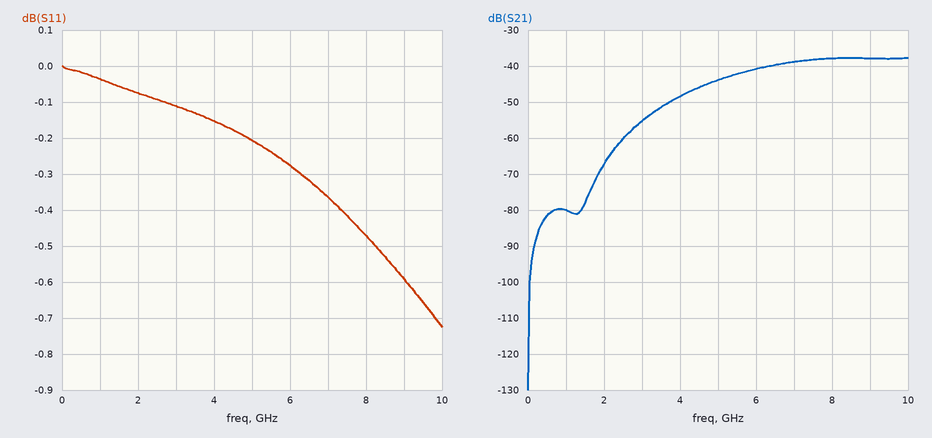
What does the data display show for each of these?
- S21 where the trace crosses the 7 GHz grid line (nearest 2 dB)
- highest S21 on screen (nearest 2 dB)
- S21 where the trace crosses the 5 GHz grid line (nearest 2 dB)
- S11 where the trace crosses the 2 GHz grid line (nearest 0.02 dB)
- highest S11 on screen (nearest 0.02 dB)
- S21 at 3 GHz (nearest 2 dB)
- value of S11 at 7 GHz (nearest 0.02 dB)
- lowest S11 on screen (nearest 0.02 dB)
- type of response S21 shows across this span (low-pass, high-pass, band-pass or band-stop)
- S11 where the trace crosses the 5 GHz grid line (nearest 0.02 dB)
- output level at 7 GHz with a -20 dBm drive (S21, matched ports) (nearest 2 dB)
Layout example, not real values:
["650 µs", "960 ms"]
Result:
["-38 dB", "-38 dB", "-44 dB", "-0.08 dB", "0.00 dB", "-56 dB", "-0.36 dB", "-0.72 dB", "high-pass", "-0.20 dB", "-58 dBm"]
